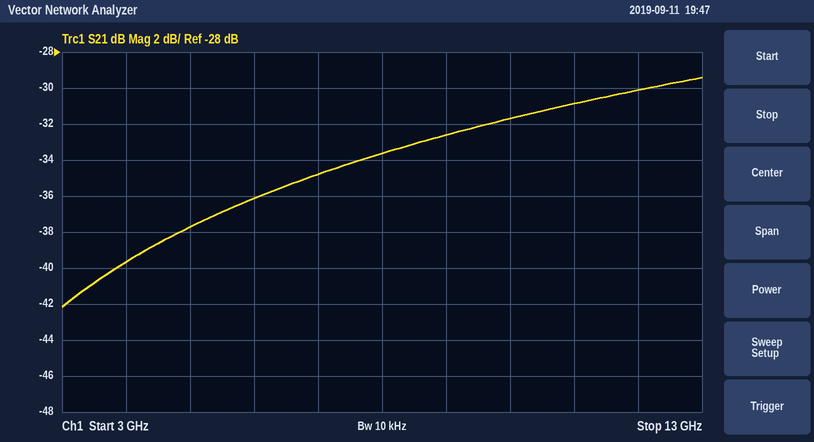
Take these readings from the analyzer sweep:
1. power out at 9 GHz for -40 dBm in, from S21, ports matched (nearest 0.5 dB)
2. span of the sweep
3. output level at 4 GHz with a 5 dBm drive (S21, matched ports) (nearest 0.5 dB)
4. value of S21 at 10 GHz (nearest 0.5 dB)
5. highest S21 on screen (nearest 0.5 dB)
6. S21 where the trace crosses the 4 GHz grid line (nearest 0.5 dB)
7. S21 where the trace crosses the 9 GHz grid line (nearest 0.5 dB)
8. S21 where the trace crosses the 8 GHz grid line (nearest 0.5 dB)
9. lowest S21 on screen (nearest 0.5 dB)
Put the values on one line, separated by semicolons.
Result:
-72.5 dBm; 10 GHz; -34.5 dBm; -31.5 dB; -29.5 dB; -39.5 dB; -32.5 dB; -33.5 dB; -42.0 dB
